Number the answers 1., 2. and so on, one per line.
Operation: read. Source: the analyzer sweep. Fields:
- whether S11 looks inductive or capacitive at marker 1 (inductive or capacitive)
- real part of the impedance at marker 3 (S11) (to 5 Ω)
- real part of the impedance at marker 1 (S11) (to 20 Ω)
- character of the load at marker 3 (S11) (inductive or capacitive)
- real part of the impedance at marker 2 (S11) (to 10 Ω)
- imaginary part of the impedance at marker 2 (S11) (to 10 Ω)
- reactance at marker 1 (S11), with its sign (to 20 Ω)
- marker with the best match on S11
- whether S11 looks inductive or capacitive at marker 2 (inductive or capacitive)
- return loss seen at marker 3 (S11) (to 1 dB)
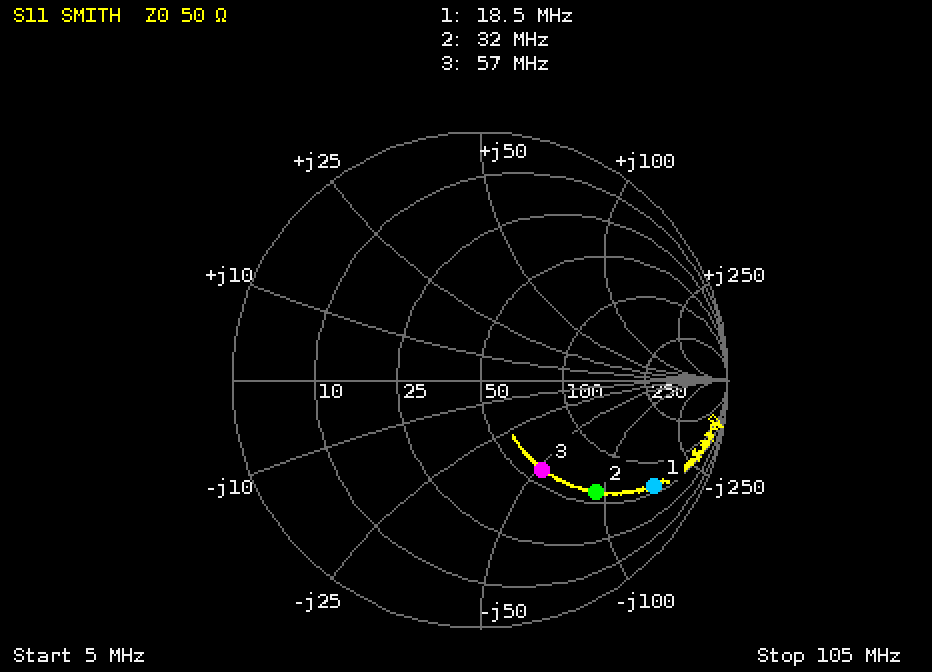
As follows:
1. capacitive
2. 60 Ω
3. 60 Ω
4. capacitive
5. 60 Ω
6. -90 Ω
7. -160 Ω
8. marker 3
9. capacitive
10. 7 dB
